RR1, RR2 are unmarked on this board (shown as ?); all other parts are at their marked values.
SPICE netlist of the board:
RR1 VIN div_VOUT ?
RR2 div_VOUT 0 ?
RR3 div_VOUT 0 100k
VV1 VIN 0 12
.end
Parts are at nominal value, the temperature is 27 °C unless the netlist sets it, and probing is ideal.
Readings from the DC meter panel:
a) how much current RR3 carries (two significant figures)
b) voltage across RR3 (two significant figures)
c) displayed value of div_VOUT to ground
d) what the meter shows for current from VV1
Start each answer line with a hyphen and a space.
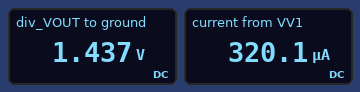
- 14 µA
- 1.4 V
- 1.437 V
- 320.1 µA
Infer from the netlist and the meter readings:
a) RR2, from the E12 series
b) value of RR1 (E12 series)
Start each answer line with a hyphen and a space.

- 4.7 kΩ
- 33 kΩ
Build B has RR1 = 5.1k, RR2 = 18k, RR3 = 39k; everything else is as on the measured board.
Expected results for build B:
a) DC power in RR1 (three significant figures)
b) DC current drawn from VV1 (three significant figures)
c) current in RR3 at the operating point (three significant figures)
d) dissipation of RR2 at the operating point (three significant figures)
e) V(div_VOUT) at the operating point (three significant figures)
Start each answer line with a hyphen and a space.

- 2.42 mW
- 689 µA
- 218 µA
- 4.00 mW
- 8.49 V
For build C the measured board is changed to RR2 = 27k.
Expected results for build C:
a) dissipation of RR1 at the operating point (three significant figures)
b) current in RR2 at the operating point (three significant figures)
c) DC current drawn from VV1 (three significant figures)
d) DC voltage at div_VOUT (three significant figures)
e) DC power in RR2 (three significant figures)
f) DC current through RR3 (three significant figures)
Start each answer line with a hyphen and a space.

- 1.61 mW
- 174 µA
- 221 µA
- 4.70 V
- 819 µW
- 47.0 µA
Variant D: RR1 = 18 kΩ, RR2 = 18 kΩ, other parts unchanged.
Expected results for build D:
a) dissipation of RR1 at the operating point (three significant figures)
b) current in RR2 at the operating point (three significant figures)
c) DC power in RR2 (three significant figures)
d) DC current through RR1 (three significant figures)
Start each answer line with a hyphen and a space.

- 2.34 mW
- 306 µA
- 1.68 mW
- 361 µA
